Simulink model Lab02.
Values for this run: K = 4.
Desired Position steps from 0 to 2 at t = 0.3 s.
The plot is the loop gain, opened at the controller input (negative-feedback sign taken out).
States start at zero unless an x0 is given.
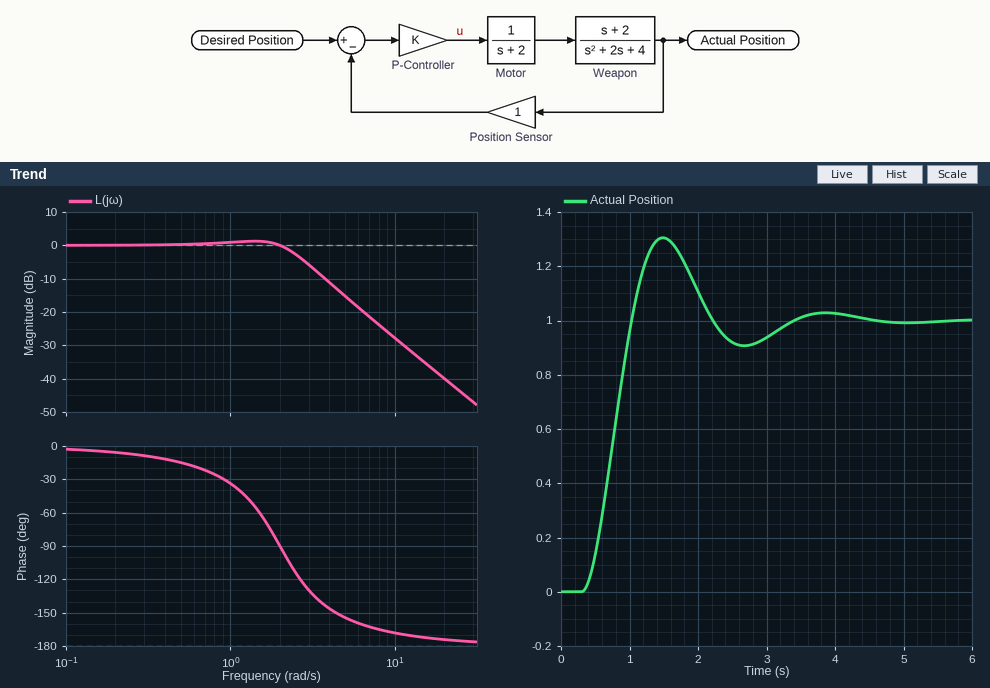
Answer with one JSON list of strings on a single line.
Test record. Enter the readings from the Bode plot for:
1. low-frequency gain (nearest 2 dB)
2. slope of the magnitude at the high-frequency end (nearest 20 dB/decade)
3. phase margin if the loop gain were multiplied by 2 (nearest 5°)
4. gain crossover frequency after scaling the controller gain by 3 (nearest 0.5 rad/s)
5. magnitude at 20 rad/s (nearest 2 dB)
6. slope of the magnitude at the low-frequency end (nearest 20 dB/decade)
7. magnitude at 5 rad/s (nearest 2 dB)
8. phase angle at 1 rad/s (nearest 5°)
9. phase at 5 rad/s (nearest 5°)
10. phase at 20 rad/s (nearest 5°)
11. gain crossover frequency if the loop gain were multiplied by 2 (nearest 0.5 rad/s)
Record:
["0 dB", "-40 dB/decade", "50°", "3.5 rad/s", "-40 dB", "0 dB/decade", "-16 dB", "-35°", "-155°", "-175°", "3.0 rad/s"]
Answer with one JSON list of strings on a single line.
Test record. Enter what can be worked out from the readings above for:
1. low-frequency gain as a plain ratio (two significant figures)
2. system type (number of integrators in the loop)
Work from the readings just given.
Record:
["1.0", "0"]
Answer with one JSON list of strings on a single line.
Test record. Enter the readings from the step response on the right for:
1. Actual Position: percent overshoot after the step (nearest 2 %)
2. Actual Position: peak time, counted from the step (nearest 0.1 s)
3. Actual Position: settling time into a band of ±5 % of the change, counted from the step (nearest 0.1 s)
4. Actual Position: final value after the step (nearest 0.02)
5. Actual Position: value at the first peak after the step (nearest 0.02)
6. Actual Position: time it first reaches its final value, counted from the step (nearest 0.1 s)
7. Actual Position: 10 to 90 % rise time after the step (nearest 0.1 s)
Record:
["30 %", "1.2 s", "2.8 s", "1.00", "1.30", "0.7 s", "0.5 s"]
